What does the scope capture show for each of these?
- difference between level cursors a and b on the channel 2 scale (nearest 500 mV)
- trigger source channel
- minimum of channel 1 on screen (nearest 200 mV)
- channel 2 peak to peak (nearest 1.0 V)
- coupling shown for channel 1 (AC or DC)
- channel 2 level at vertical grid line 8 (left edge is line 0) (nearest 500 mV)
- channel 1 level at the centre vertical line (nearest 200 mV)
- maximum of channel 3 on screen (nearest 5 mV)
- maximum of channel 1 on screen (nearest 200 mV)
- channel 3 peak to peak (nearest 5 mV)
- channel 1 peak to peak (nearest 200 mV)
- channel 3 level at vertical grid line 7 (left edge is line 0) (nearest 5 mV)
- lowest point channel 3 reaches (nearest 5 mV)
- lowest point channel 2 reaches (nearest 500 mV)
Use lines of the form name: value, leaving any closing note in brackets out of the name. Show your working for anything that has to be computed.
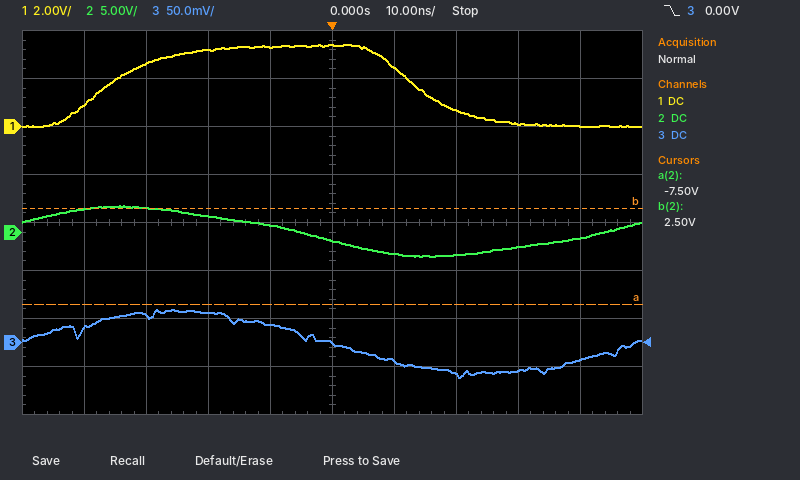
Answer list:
difference between level cursors a and b on the channel 2 scale: 10.0 V
trigger source channel: channel 3
minimum of channel 1 on screen: 0.0 V
channel 2 peak to peak: 5.0 V
coupling shown for channel 1: DC
channel 2 level at vertical grid line 8 (left edge is line 0): -1.5 V
channel 1 level at the centre vertical line: 3.4 V
maximum of channel 3 on screen: 35 mV
maximum of channel 1 on screen: 3.4 V
channel 3 peak to peak: 35 mV − (-35 mV) = 70 mV
channel 1 peak to peak: 3.4 V − (0.0 V) = 3.4 V
channel 3 level at vertical grid line 7 (left edge is line 0): -35 mV
lowest point channel 3 reaches: -35 mV
lowest point channel 2 reaches: -2.5 V
